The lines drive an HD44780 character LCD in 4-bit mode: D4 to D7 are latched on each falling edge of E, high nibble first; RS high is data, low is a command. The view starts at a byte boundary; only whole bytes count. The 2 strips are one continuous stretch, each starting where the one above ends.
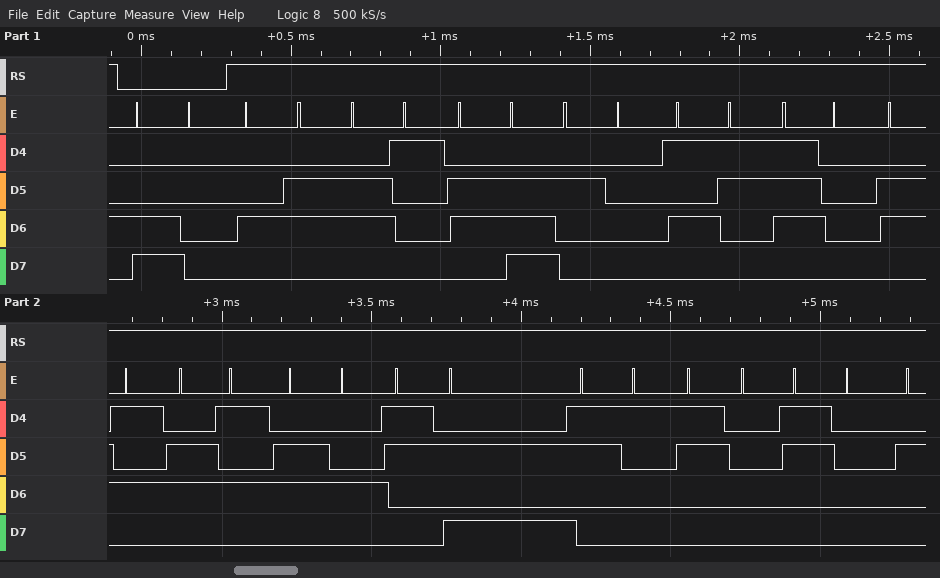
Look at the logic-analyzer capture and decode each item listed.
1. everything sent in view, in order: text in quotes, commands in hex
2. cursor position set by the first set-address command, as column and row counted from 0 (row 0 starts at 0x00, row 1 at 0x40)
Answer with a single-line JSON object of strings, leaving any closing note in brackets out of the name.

{"everything sent in view, in order: text in quotes, commands in hex": "0xC0 \"Fan Speed:100\"", "cursor position set by the first set-address command, as column and row counted from 0": "column 0, row 1"}
